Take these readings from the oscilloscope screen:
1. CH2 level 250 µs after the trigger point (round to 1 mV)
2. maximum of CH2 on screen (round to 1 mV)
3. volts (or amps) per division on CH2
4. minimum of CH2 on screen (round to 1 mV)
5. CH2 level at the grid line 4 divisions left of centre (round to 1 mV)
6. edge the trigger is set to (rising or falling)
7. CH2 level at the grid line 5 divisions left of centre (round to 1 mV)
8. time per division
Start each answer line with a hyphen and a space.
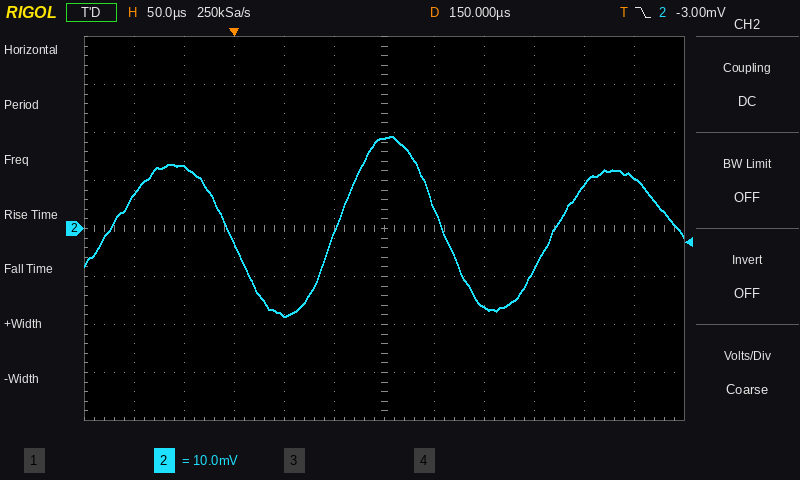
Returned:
- -16 mV
- 19 mV
- 10 mV
- -18 mV
- 13 mV
- falling
- 7 mV
- 50 µs
